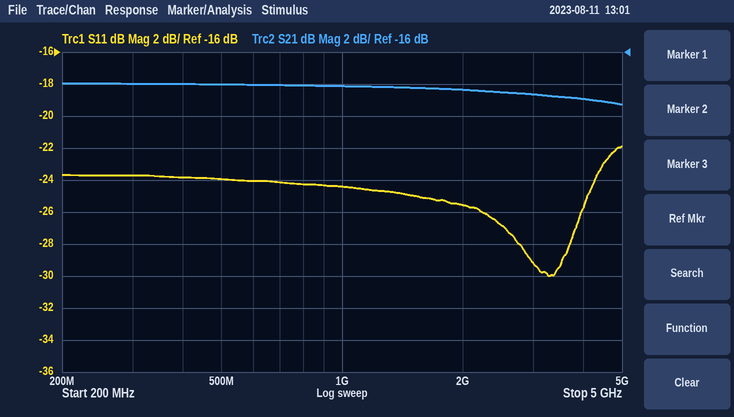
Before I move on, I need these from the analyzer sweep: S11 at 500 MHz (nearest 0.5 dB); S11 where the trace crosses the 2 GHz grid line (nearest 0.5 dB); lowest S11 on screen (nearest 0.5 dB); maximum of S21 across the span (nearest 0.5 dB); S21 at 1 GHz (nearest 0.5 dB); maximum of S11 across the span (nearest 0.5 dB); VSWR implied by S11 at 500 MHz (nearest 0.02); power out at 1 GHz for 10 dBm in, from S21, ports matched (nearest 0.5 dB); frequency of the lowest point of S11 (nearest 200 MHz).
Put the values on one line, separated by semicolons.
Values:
-24.0 dB; -25.5 dB; -30.0 dB; -18.0 dB; -18.0 dB; -22.0 dB; 1.14; -8.0 dBm; 3.2 GHz
